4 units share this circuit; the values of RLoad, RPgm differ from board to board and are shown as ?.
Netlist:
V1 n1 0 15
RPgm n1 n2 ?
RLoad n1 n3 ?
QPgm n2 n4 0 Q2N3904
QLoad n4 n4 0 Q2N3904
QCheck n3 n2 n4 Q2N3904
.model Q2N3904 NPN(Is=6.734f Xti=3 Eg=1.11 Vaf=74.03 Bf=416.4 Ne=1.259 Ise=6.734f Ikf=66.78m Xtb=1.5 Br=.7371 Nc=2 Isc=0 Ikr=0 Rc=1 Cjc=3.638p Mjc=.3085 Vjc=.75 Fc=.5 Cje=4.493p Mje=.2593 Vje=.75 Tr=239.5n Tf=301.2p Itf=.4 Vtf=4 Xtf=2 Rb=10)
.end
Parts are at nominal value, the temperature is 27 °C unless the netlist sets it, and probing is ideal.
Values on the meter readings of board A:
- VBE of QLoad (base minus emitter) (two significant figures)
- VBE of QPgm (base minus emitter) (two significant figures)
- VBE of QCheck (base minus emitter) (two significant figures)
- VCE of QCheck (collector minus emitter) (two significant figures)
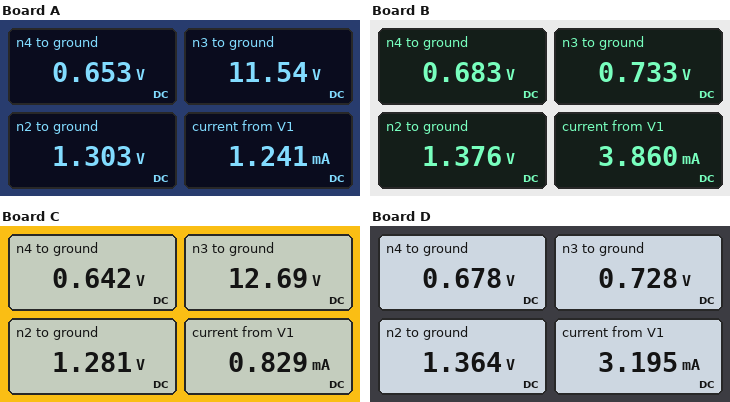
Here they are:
650 mV
650 mV
650 mV
11 V
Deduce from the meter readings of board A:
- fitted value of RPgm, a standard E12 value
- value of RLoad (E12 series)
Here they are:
22 kΩ
5.6 kΩ
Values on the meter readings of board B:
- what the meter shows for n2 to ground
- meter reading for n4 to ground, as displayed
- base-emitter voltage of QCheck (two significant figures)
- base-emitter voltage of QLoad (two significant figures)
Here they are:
1.376 V
0.683 V
690 mV
680 mV
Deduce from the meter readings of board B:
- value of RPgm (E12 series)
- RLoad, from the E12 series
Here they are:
5.6 kΩ
10 kΩ
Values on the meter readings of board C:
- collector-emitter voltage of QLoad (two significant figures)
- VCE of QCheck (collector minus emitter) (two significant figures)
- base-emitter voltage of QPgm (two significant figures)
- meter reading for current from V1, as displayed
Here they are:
640 mV
12 V
640 mV
0.829 mA
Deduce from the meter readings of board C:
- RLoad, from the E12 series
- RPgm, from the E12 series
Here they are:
5.6 kΩ
33 kΩ
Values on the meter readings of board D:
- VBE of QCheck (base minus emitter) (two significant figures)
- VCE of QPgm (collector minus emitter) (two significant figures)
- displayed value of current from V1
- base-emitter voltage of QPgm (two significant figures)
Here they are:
690 mV
1.4 V
3.195 mA
680 mV
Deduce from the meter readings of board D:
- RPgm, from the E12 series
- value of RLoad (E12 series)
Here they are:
6.8 kΩ
12 kΩ
